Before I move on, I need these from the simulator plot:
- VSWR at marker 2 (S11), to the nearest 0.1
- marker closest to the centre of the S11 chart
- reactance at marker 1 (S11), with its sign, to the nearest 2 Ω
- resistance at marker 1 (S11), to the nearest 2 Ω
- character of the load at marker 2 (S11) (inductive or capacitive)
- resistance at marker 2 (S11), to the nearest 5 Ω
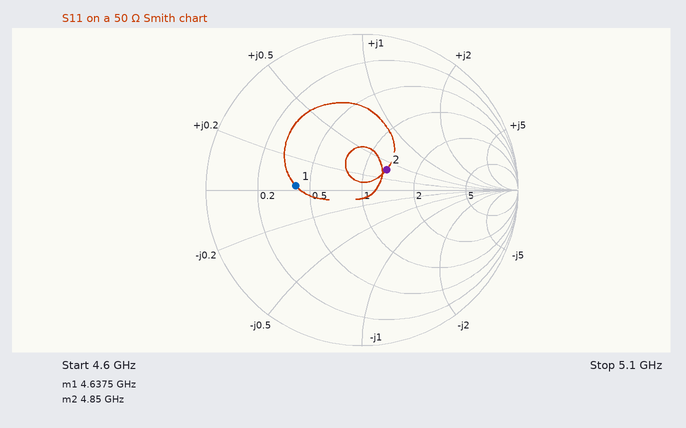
1.5
marker 2
+2 Ω
20 Ω
inductive
65 Ω
